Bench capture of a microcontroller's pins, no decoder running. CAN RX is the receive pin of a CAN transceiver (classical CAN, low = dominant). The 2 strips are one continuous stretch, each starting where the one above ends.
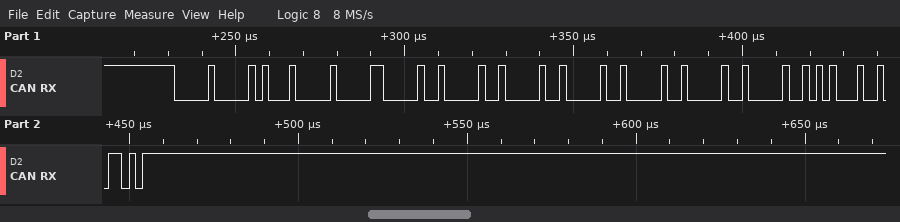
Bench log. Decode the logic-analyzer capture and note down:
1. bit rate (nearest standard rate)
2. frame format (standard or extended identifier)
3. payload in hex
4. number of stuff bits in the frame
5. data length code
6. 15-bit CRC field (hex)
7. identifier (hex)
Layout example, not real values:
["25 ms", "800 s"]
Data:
["500 kbit/s", "standard", "01 01 01 01 01 01 01 01", "11", "8", "0x2896", "0x001"]
